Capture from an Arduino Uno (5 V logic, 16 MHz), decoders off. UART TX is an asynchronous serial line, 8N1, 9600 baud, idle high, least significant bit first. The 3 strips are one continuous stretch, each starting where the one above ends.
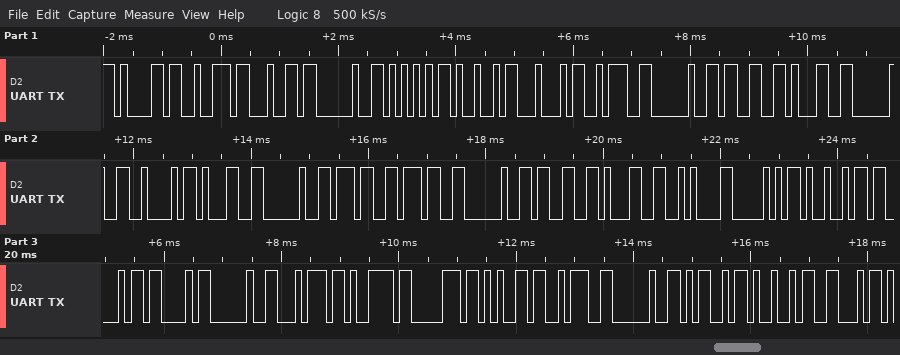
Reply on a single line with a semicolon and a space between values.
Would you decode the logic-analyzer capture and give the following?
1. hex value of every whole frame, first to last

61 72 64 20 55 49 44 3A 20 33 31 20 42 31 20 37 37 20 33 31 0A 50 49 43 43 20 74 79 70 65 3A 20 4D 49 46
